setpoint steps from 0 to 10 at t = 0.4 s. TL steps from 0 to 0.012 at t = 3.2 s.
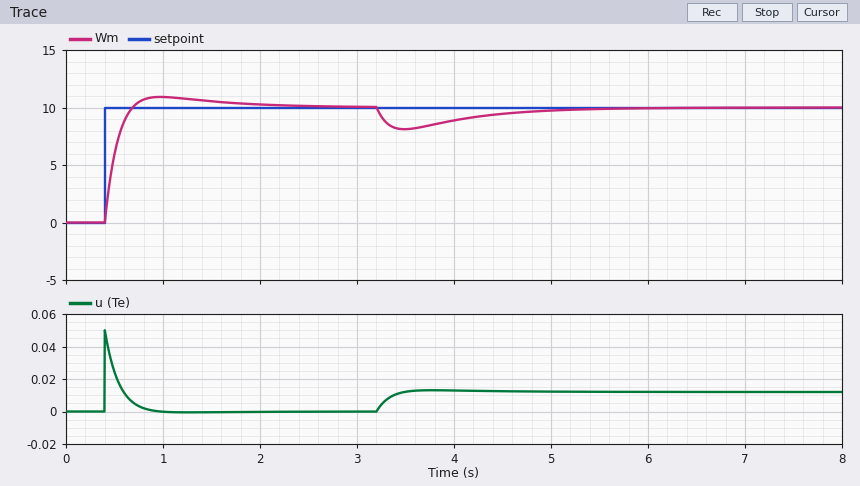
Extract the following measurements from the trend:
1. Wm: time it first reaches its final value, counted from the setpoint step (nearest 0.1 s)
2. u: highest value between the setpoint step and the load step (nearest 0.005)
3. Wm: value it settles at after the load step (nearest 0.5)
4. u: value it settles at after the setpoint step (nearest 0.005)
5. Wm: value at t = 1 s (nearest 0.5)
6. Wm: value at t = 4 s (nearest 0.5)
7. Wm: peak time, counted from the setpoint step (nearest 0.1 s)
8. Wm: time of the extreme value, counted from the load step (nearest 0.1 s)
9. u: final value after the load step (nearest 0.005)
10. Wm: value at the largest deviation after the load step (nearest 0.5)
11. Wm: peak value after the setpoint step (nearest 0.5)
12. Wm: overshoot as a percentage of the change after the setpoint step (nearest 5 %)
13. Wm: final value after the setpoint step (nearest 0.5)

0.3 s
0.050
10.0
0.000
11.0
9.0
0.6 s
0.3 s
0.010
8.0
11.0
10 %
10.0
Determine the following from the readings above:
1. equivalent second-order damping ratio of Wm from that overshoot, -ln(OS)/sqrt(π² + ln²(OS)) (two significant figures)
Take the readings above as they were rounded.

0.59
